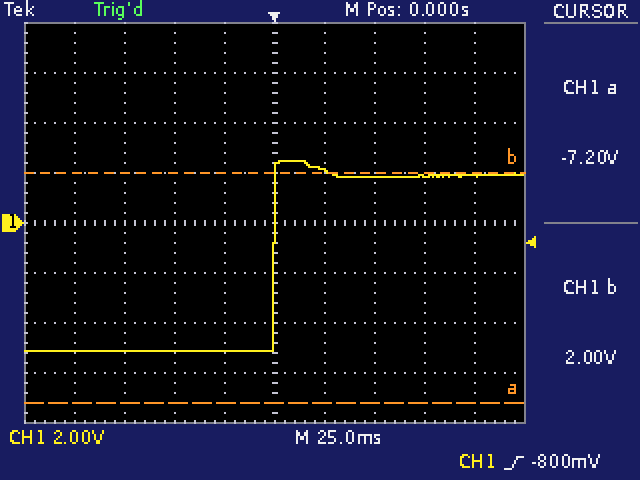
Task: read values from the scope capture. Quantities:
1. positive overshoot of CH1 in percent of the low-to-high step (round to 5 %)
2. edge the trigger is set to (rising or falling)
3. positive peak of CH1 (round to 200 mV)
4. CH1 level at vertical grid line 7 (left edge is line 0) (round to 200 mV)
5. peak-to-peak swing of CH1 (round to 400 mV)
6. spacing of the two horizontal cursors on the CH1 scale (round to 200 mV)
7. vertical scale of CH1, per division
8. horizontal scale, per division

10 %
rising
2.4 V
1.8 V
7.6 V
9.2 V
2 V
25 ms
